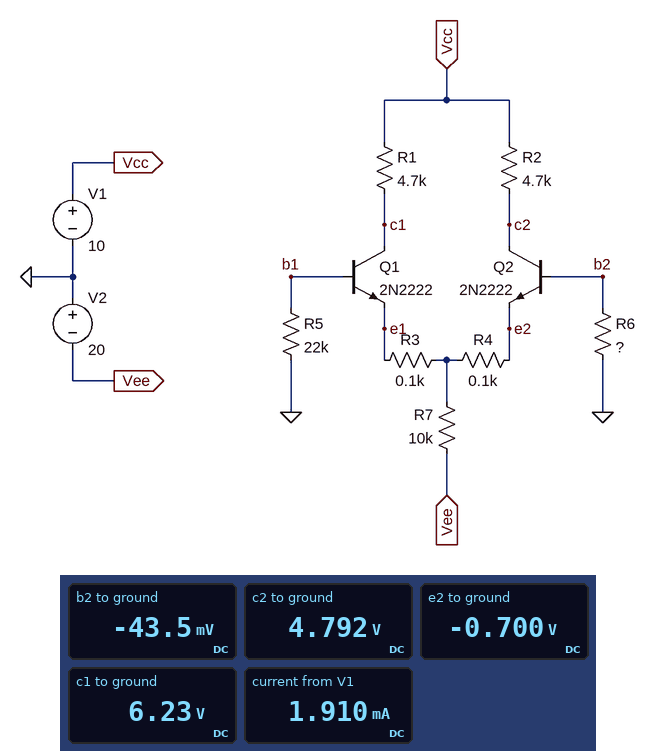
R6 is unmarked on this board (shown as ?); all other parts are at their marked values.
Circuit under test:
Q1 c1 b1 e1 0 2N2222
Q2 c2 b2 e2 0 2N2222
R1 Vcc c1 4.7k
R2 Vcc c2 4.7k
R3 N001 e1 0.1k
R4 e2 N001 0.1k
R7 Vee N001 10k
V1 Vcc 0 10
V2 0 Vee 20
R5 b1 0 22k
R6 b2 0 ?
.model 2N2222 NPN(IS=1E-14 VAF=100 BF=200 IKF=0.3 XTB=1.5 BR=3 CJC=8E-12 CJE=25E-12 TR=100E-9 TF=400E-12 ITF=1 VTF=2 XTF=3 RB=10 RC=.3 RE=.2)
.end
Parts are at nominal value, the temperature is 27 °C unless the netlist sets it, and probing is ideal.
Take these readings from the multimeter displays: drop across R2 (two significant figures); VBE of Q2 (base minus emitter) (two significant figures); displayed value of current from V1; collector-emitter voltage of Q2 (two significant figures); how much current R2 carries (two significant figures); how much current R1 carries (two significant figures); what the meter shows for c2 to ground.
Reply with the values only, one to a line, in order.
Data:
5.2 V
660 mV
1.910 mA
5.5 V
1.1 mA
800 µA
4.792 V
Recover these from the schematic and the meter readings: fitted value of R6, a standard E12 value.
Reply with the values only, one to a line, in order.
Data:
8.2 kΩ
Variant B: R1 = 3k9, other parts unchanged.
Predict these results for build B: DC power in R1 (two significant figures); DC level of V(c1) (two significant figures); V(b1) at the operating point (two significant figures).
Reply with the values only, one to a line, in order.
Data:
2.5 mW
6.9 V
-83 mV
